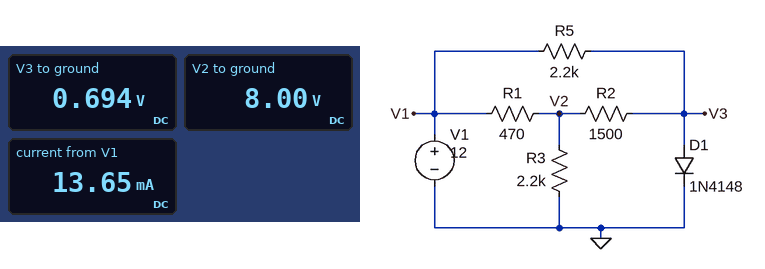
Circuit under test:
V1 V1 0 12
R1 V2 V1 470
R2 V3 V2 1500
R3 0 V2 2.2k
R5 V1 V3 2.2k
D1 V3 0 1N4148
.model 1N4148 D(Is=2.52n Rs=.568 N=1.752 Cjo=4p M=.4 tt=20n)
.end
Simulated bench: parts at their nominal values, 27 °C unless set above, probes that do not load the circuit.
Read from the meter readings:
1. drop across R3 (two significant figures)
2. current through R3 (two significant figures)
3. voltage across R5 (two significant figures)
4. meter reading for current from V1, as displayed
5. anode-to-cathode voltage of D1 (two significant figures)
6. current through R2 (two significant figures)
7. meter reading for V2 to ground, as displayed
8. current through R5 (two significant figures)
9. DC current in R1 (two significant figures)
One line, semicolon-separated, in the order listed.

8.0 V; 3.6 mA; 11 V; 13.65 mA; 690 mV; 4.9 mA; 8.00 V; 5.1 mA; 8.5 mA
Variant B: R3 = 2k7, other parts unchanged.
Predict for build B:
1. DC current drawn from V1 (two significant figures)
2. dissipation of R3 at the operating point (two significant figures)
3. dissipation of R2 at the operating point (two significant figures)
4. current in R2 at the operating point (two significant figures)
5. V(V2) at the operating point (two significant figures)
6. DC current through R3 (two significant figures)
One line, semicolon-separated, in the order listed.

13 mA; 25 mW; 38 mW; 5.0 mA; 8.2 V; 3.0 mA
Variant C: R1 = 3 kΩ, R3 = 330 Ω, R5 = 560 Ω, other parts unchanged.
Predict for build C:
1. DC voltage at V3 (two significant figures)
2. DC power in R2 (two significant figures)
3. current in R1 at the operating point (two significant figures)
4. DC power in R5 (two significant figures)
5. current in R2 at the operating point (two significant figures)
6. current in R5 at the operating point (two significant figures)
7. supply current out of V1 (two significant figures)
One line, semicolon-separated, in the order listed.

730 mV; 97 µW; 3.6 mA; 230 mW; 250 µA; 20 mA; 24 mA
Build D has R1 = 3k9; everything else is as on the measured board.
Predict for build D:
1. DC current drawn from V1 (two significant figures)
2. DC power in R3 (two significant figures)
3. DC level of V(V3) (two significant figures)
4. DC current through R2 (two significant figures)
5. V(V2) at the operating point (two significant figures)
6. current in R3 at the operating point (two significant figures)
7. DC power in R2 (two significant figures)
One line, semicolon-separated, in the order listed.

7.6 mA; 3.0 mW; 670 mV; 1.3 mA; 2.6 V; 1.2 mA; 2.4 mW
